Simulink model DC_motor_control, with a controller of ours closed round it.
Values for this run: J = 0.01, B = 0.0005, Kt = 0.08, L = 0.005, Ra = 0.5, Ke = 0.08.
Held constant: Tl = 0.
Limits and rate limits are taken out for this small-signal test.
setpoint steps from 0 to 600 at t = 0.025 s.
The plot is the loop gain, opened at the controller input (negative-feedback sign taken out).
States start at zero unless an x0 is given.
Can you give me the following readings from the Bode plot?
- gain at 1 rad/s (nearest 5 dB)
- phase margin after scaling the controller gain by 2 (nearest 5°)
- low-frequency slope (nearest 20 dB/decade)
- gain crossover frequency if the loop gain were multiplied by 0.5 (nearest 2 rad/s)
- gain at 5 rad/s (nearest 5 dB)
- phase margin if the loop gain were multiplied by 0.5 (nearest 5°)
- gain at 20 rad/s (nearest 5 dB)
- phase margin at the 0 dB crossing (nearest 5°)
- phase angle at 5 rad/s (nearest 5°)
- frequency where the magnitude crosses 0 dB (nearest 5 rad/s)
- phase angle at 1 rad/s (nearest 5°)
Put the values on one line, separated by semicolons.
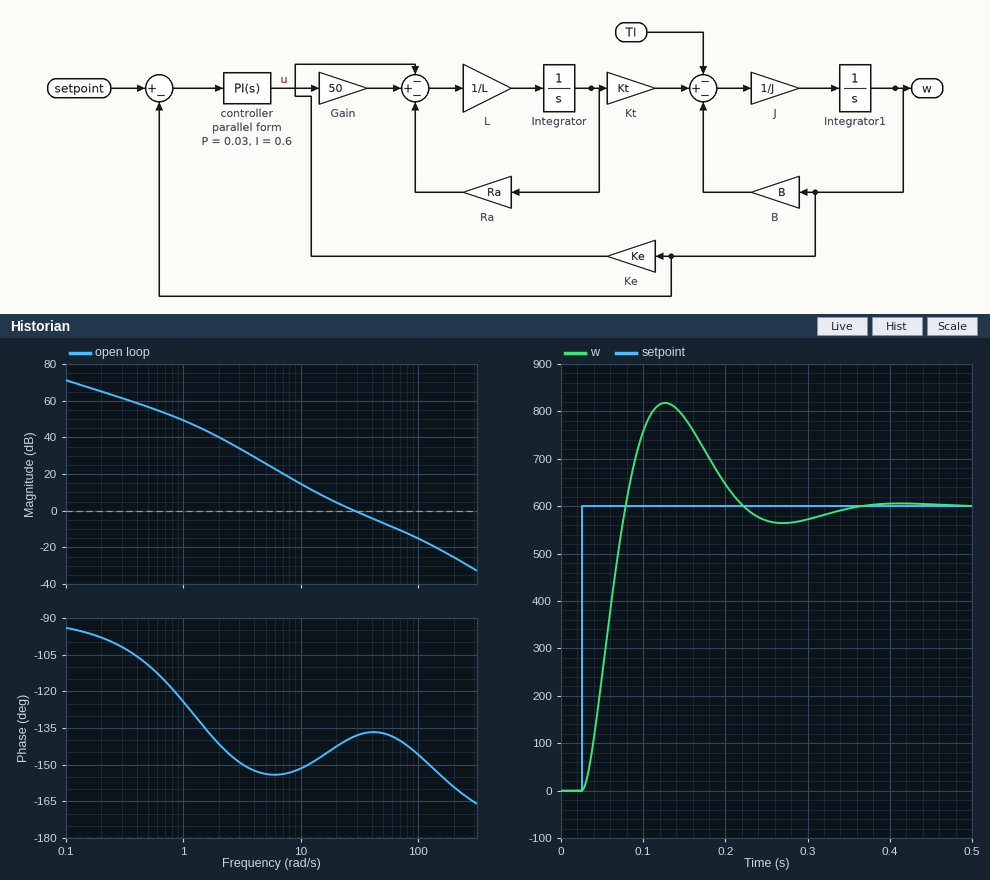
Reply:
50 dB; 45°; -20 dB/decade; 18 rad/s; 25 dB; 35°; 5 dB; 40°; -155°; 30 rad/s; -125°
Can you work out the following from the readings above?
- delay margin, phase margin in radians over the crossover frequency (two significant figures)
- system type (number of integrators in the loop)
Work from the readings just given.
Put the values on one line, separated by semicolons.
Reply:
0.023 s; 1
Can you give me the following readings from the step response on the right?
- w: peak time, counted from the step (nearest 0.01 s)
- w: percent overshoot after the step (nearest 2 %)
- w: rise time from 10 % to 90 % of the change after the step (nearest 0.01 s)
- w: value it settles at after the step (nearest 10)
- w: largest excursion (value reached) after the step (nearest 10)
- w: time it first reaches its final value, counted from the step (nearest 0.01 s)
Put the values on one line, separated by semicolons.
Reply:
0.10 s; 36 %; 0.04 s; 600; 820; 0.05 s
